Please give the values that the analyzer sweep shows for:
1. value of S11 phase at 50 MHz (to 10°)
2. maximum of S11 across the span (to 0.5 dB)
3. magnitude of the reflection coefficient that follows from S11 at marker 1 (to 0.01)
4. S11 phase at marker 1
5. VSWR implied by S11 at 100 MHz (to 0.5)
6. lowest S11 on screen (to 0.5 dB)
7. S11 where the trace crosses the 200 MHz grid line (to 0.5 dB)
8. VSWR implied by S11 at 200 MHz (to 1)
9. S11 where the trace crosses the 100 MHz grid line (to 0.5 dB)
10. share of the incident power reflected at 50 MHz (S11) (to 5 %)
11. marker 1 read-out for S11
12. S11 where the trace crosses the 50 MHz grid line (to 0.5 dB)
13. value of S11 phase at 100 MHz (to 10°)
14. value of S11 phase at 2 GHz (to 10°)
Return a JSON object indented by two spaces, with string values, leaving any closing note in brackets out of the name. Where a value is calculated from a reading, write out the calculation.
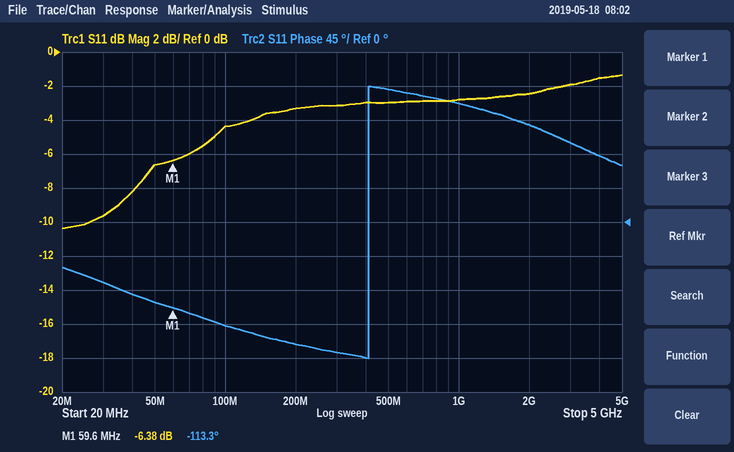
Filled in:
{
  "value of S11 phase at 50 MHz": "-110°",
  "maximum of S11 across the span": "-1.5 dB",
  "magnitude of the reflection coefficient that follows from S11 at marker 1": "10^(-6.38/20) ≈ 0.48",
  "S11 phase at marker 1": "-113.3°",
  "VSWR implied by S11 at 100 MHz": "|Γ| = 10^(-4.5/20) = 0.5957; VSWR = (1 + 0.5957)/(1 − 0.5957) ≈ 4.0",
  "lowest S11 on screen": "-10.5 dB",
  "S11 where the trace crosses the 200 MHz grid line": "-3.5 dB",
  "VSWR implied by S11 at 200 MHz": "|Γ| = 10^(-3.5/20) = 0.6683; VSWR = (1 + 0.6683)/(1 − 0.6683) ≈ 5",
  "S11 where the trace crosses the 100 MHz grid line": "-4.5 dB",
  "share of the incident power reflected at 50 MHz (S11)": "10^(-6.5/10) ≈ 22.4 %, so 20 % to the nearest 5 %",
  "marker 1 read-out for S11": "-6.38 dB",
  "S11 where the trace crosses the 50 MHz grid line": "-6.5 dB",
  "value of S11 phase at 100 MHz": "-140°",
  "value of S11 phase at 2 GHz": "130°"
}
